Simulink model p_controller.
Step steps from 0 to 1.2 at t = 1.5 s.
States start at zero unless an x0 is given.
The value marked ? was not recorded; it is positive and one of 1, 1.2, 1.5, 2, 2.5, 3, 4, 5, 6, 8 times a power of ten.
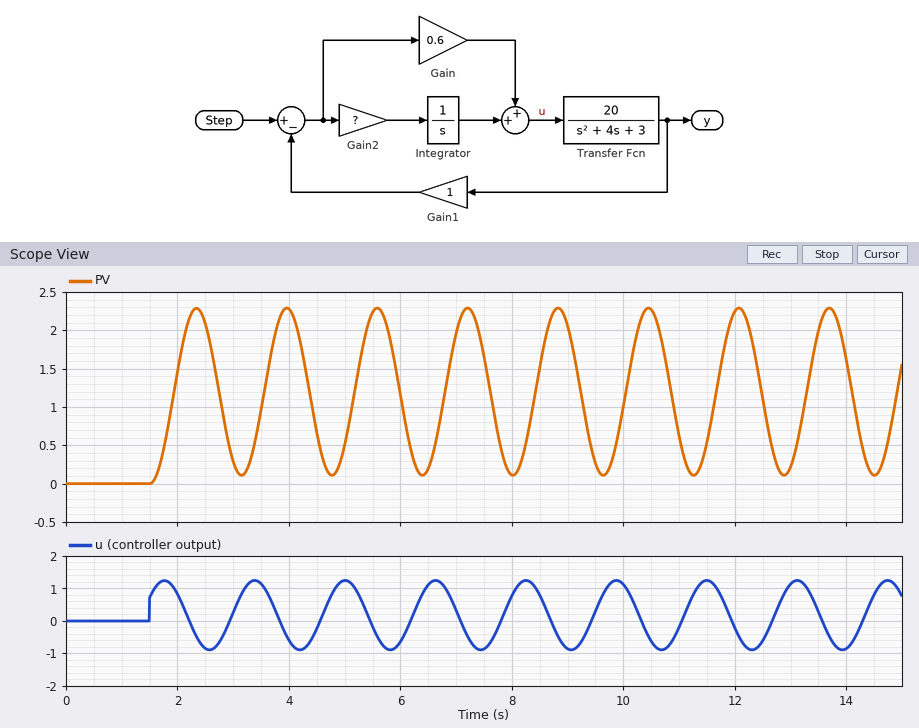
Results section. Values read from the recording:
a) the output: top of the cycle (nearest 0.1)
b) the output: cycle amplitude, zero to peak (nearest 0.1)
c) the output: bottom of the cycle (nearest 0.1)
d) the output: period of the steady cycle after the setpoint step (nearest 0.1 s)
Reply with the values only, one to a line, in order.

2.3
1.1
0.1
1.6 s
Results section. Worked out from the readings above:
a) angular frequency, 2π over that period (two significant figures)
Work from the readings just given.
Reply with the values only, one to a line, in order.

3.9 rad/s
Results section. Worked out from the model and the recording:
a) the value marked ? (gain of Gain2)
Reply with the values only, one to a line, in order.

3
